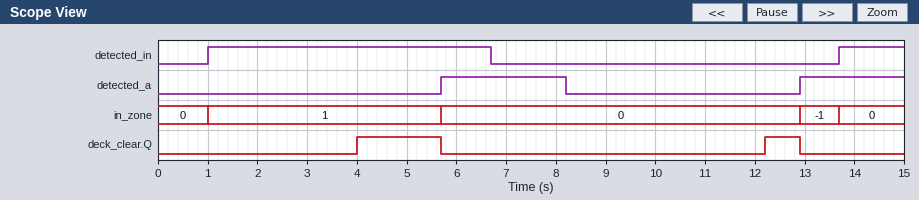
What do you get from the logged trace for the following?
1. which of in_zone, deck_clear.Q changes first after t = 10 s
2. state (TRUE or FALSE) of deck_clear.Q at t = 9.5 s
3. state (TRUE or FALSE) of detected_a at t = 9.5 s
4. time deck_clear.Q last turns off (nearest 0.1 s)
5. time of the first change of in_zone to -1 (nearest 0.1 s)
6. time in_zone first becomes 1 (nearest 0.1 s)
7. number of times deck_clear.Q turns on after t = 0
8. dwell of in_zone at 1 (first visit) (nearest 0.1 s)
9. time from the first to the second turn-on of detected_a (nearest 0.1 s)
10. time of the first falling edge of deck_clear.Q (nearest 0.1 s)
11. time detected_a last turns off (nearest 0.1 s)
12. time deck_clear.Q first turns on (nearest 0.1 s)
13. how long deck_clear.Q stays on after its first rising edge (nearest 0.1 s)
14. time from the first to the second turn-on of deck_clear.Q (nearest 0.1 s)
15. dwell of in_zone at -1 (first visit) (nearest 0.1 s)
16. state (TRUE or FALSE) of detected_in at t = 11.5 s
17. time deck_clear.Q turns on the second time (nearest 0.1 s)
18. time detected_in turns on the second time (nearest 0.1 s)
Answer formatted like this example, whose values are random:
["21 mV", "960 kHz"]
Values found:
["deck_clear.Q", "FALSE", "FALSE", "12.9 s", "12.9 s", "1.0 s", "2", "4.7 s", "7.2 s", "5.7 s", "8.2 s", "4.0 s", "1.7 s", "8.2 s", "0.8 s", "FALSE", "12.2 s", "13.7 s"]
